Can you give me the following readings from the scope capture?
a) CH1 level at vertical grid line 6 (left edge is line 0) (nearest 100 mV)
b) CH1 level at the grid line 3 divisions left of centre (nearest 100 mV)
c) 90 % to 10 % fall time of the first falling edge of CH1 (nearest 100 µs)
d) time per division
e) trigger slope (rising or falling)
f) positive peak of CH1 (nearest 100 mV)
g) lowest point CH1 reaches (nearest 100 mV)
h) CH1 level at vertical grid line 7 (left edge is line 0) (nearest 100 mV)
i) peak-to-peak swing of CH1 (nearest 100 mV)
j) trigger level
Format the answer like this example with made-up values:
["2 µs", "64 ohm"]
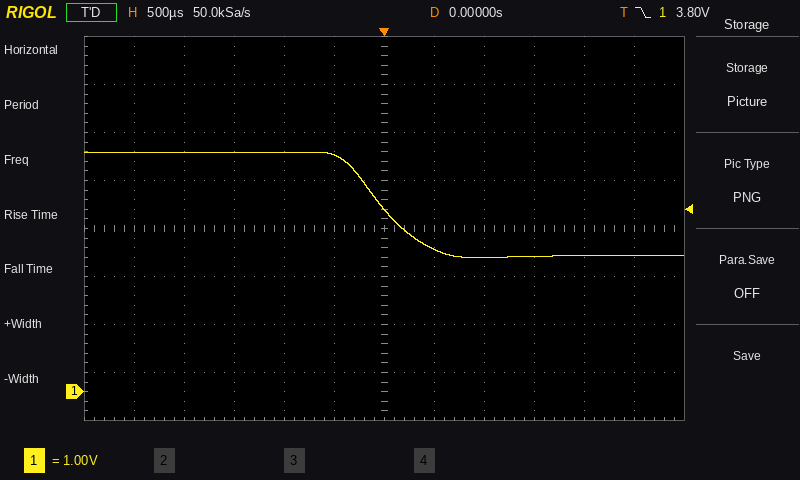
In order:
["3.8 V", "5.0 V", "800 µs", "500 µs", "falling", "5.0 V", "2.8 V", "3.0 V", "2.2 V", "3.80 V"]
